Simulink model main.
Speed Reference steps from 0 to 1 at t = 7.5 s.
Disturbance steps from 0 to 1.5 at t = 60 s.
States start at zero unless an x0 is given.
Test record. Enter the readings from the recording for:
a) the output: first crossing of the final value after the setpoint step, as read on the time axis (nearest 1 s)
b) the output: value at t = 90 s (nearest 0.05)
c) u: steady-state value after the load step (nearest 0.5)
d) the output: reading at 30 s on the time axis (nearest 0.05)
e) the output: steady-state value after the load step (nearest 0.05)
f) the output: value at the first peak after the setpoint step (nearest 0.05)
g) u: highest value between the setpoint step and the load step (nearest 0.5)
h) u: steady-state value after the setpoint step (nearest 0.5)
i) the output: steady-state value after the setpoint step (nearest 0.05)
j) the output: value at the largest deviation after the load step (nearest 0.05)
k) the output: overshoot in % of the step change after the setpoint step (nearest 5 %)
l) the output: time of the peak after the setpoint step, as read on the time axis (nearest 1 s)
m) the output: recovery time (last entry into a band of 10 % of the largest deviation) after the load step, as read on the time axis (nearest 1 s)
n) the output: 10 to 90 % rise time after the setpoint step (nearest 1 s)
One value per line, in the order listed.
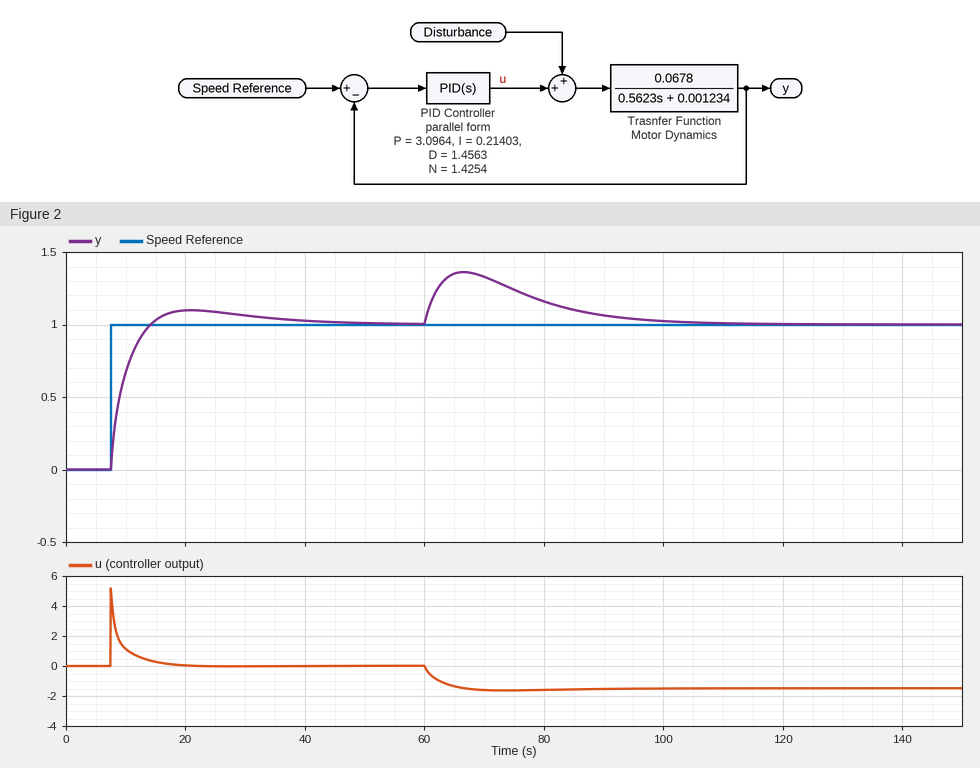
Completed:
14 s
1.05
-1.5
1.05
1.00
1.10
5.0
0.0
1.00
1.35
10 %
21 s
96 s
5 s
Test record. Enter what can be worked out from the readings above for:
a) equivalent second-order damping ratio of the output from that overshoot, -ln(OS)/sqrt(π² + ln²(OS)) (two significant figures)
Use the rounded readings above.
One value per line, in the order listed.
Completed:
0.59
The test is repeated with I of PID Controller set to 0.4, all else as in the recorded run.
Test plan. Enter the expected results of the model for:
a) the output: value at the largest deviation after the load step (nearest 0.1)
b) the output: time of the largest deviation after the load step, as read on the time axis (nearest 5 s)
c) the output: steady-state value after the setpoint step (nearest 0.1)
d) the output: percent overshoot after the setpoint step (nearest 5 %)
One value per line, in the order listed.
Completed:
1.3
65 s
1.0
15 %
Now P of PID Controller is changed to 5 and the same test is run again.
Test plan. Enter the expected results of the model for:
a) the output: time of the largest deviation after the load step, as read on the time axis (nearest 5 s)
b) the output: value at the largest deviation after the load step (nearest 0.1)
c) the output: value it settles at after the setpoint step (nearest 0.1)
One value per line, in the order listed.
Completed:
65 s
1.3
1.0
